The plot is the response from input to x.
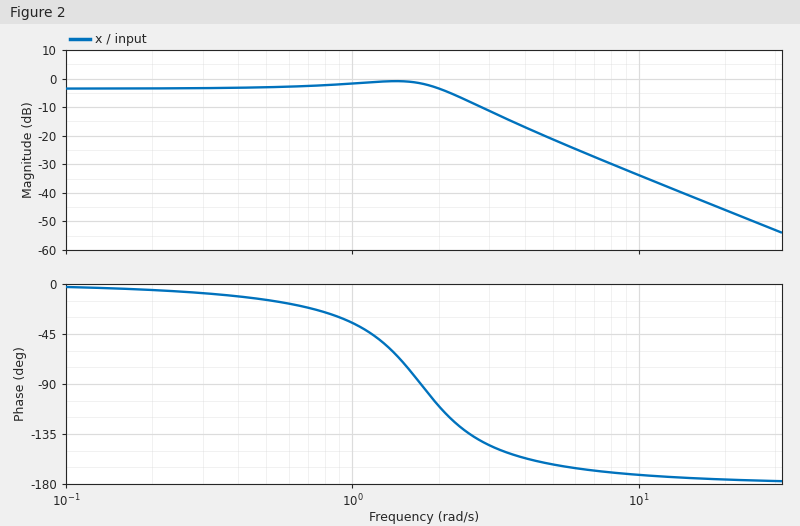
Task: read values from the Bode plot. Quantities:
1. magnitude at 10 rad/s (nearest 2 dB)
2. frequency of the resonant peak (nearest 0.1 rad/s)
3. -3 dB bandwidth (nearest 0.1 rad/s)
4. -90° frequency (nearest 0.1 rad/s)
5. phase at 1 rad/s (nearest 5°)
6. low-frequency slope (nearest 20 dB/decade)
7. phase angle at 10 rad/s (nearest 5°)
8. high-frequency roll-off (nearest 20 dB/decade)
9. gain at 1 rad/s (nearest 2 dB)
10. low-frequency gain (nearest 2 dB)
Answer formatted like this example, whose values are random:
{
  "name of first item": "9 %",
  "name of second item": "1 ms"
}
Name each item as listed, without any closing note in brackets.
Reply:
{
  "magnitude at 10 rad/s": "-34 dB",
  "frequency of the resonant peak": "1.4 rad/s",
  "-3 dB bandwidth": "2.4 rad/s",
  "-90° frequency": "1.7 rad/s",
  "phase at 1 rad/s": "-35°",
  "low-frequency slope": "0 dB/decade",
  "phase angle at 10 rad/s": "-170°",
  "high-frequency roll-off": "-40 dB/decade",
  "gain at 1 rad/s": "-2 dB",
  "low-frequency gain": "-4 dB"
}
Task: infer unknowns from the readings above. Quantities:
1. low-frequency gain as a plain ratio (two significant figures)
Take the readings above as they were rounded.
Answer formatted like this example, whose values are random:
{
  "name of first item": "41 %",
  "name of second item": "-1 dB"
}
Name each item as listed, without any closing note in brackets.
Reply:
{
  "low-frequency gain as a plain ratio": "0.63"
}
